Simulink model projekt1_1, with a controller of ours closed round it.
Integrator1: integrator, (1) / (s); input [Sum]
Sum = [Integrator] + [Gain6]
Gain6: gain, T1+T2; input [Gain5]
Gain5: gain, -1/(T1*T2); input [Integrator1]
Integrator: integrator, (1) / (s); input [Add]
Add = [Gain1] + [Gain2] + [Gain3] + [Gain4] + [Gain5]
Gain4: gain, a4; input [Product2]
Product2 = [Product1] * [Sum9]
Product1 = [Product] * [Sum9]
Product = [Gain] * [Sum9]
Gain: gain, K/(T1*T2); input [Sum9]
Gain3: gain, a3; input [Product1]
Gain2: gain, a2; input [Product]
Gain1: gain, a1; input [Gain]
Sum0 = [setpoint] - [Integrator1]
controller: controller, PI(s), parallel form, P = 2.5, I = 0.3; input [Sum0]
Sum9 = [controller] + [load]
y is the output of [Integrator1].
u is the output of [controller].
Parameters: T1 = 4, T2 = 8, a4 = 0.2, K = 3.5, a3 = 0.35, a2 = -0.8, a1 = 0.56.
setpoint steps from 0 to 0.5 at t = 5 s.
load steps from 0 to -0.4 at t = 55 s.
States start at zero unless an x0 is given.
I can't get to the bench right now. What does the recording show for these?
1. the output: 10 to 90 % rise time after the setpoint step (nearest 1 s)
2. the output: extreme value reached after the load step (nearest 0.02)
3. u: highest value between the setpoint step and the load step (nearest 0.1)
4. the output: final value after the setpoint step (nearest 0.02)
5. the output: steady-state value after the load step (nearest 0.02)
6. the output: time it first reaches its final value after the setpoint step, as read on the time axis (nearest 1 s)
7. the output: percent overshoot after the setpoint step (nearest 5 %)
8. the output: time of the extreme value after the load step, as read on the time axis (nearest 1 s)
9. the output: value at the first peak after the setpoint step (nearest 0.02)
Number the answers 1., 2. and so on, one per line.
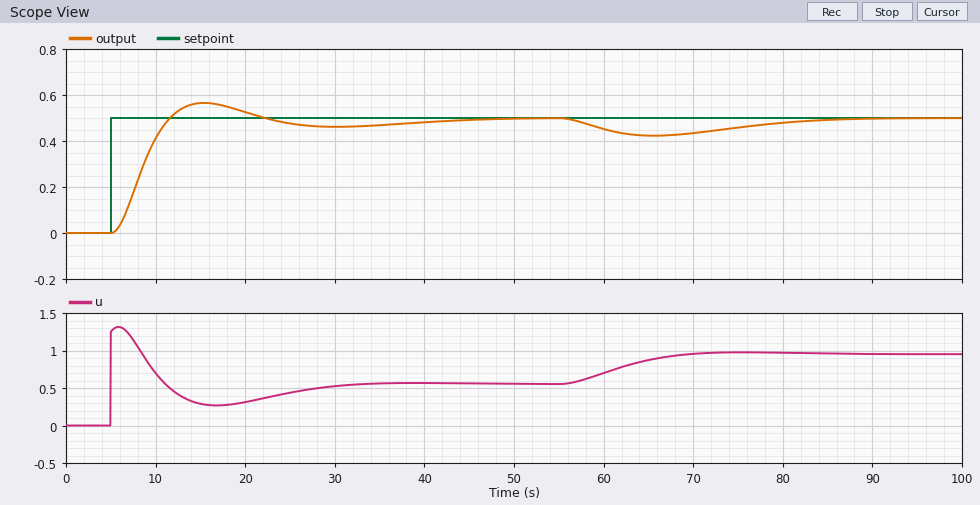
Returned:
1. 4 s
2. 0.42
3. 1.3
4. 0.50
5. 0.50
6. 12 s
7. 15 %
8. 66 s
9. 0.56
